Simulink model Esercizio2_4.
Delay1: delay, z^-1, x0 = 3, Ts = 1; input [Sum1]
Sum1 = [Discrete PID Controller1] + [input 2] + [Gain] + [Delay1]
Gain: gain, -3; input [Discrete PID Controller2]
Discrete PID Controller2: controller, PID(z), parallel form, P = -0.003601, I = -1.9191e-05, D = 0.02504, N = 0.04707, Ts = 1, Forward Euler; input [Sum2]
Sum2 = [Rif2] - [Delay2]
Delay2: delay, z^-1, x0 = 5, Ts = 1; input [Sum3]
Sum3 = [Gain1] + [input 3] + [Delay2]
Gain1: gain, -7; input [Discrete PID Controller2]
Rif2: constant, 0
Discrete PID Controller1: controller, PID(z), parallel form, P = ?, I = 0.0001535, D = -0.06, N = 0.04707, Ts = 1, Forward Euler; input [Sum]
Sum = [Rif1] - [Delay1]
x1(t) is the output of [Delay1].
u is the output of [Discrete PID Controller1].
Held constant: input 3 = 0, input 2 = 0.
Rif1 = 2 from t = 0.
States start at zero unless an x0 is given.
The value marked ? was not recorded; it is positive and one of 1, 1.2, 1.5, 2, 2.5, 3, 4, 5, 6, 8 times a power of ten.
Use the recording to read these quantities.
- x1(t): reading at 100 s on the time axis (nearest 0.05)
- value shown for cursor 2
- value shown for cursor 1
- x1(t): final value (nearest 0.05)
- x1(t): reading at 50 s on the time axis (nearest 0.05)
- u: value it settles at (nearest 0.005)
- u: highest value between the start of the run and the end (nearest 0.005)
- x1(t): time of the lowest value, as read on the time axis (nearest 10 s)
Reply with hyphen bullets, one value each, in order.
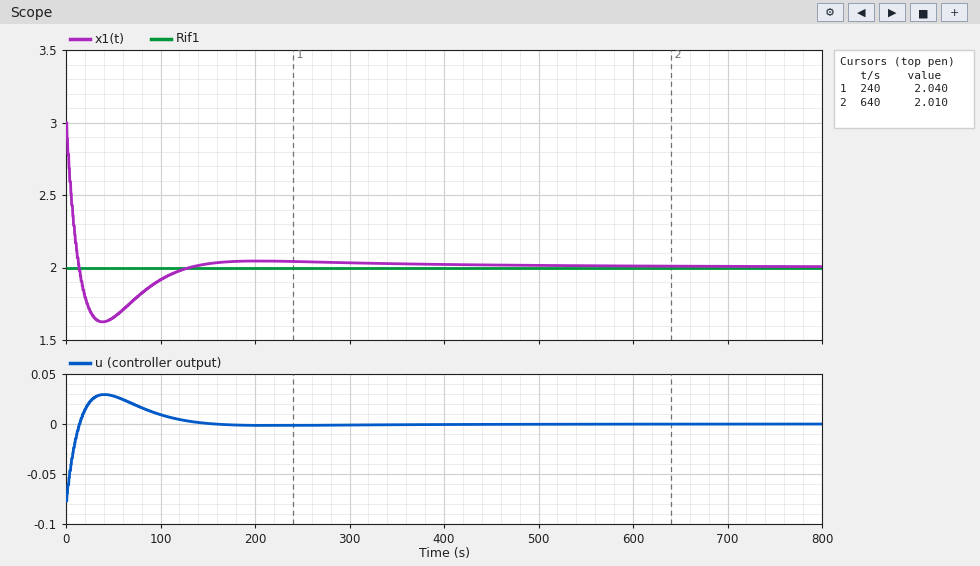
- 1.90
- 2.010
- 2.040
- 2.00
- 1.65
- 0.000
- 0.030
- 40 s
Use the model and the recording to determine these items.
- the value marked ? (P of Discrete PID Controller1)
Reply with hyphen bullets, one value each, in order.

- 0.08
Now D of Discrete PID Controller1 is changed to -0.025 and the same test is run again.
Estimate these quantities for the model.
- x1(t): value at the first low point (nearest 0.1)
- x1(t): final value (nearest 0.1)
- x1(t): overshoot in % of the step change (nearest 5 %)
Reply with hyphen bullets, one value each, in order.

- 1.6
- 2.0
- 35 %
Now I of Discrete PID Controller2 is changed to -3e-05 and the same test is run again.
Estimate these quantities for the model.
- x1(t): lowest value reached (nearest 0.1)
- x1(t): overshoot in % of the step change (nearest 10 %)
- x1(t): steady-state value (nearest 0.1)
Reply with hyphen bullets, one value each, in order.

- 1.6
- 40 %
- 2.0
